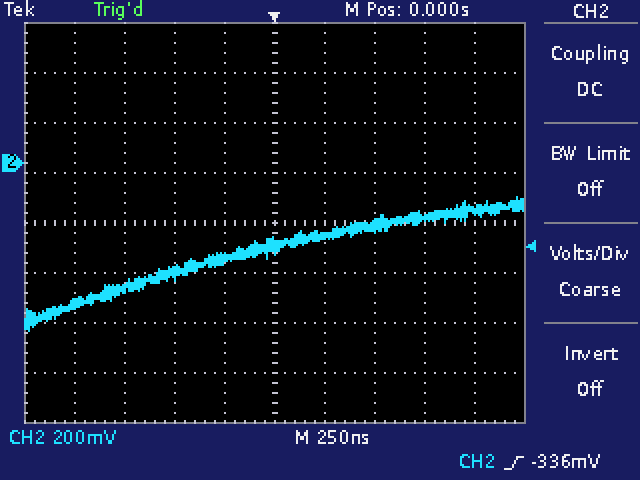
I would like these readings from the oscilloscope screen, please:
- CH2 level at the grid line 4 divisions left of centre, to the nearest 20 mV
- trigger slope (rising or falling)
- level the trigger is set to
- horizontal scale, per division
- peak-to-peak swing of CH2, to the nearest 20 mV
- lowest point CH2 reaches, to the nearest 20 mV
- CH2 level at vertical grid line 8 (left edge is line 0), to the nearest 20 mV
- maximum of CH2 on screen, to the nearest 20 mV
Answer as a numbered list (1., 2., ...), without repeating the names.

1. -560 mV
2. rising
3. -336 mV
4. 250 ns
5. 540 mV
6. -680 mV
7. -220 mV
8. -140 mV
